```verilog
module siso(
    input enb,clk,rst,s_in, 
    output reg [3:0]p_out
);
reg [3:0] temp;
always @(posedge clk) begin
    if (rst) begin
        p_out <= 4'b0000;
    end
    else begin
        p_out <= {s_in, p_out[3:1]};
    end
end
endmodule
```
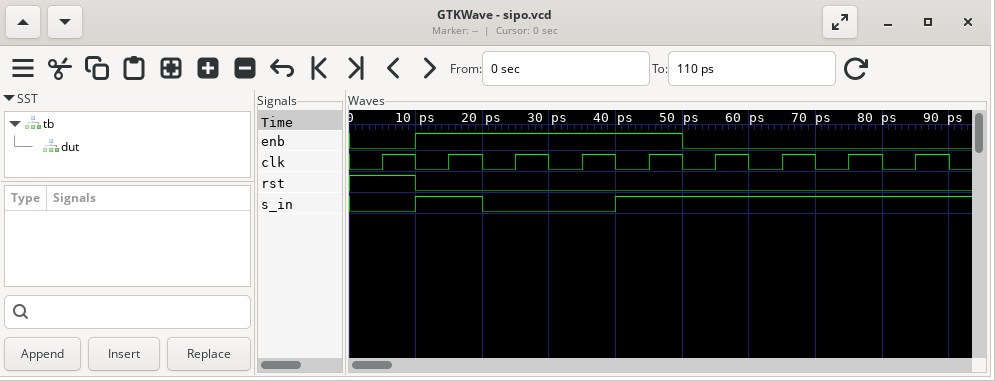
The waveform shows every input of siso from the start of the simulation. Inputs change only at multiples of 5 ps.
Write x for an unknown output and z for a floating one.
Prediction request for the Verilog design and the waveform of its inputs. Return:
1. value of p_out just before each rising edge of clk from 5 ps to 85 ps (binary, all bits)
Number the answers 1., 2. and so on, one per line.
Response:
1. x, 0000, 1000, 0100, 0010, 1001, 1100, 1110, 1111
